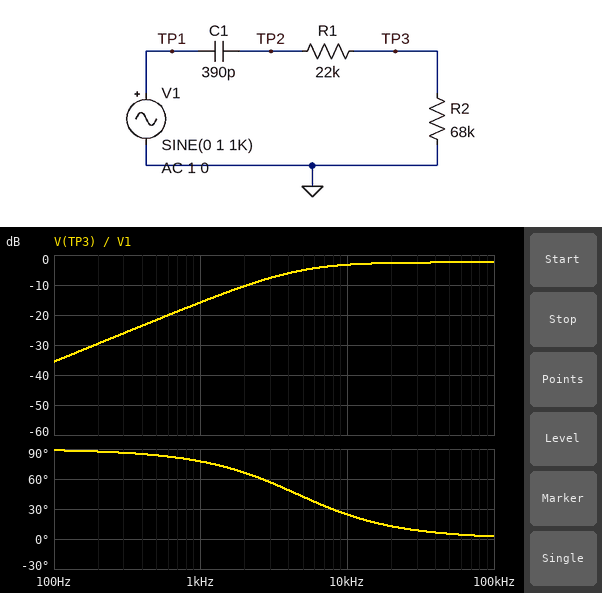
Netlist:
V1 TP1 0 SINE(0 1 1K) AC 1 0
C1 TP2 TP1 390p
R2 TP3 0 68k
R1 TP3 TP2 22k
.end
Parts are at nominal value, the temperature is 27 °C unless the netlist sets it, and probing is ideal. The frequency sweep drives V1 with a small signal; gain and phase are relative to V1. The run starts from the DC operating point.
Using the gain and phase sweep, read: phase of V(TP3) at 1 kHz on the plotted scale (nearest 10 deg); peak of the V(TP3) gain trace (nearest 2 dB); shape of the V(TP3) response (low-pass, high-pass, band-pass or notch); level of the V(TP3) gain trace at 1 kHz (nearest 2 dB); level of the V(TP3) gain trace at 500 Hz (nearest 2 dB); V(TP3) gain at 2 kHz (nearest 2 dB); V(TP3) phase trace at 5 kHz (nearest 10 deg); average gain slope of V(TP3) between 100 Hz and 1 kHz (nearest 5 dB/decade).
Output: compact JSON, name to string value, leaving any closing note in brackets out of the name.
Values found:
{"phase of V(TP3) at 1 kHz on the plotted scale": "80 deg", "peak of the V(TP3) gain trace": "-2 dB", "shape of the V(TP3) response": "high-pass", "level of the V(TP3) gain trace at 1 kHz": "-16 dB", "level of the V(TP3) gain trace at 500 Hz": "-22 dB", "V(TP3) gain at 2 kHz": "-10 dB", "V(TP3) phase trace at 5 kHz": "40 deg", "average gain slope of V(TP3) between 100 Hz and 1 kHz": "20 dB/decade"}
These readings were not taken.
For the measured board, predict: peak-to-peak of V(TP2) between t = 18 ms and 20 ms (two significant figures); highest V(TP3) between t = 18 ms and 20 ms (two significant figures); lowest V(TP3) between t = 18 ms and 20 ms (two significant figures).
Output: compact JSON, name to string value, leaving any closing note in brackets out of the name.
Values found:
{"peak-to-peak of V(TP2) between t = 18 ms and 20 ms": "430 mV", "highest V(TP3) between t = 18 ms and 20 ms": "160 mV", "lowest V(TP3) between t = 18 ms and 20 ms": "-160 mV"}
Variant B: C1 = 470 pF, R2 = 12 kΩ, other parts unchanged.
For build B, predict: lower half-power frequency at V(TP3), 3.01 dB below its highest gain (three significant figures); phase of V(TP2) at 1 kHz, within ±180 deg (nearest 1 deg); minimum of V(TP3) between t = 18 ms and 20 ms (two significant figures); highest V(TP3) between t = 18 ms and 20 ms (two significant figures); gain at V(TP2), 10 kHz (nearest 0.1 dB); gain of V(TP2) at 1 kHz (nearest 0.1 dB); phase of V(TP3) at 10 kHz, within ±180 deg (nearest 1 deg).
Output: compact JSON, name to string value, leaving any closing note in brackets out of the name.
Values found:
{"lower half-power frequency at V(TP3), 3.01 dB below its highest gain": "9.96 kHz", "phase of V(TP2) at 1 kHz, within ±180 deg": "84 deg", "minimum of V(TP3) between t = 18 ms and 20 ms": "-35 mV", "highest V(TP3) between t = 18 ms and 20 ms": "35 mV", "gain at V(TP2), 10 kHz": "-3.0 dB", "gain of V(TP2) at 1 kHz": "-20.0 dB", "phase of V(TP3) at 10 kHz, within ±180 deg": "45 deg"}
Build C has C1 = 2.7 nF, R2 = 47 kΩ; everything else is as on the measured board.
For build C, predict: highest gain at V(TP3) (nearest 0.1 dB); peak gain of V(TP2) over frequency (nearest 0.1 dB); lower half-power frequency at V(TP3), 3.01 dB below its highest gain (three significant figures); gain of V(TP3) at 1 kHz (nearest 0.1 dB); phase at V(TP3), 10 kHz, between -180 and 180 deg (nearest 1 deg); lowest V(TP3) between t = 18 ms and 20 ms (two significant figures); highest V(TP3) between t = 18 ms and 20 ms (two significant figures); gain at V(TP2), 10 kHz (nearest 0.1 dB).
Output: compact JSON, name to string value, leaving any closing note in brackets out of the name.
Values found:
{"highest gain at V(TP3)": "-3.3 dB", "peak gain of V(TP2) over frequency": "0 dB", "lower half-power frequency at V(TP3), 3.01 dB below its highest gain": "854 Hz", "gain of V(TP3) at 1 kHz": "-5.7 dB", "phase at V(TP3), 10 kHz, between -180 and 180 deg": "5 deg", "lowest V(TP3) between t = 18 ms and 20 ms": "-520 mV", "highest V(TP3) between t = 18 ms and 20 ms": "520 mV", "gain at V(TP2), 10 kHz": "0 dB"}
